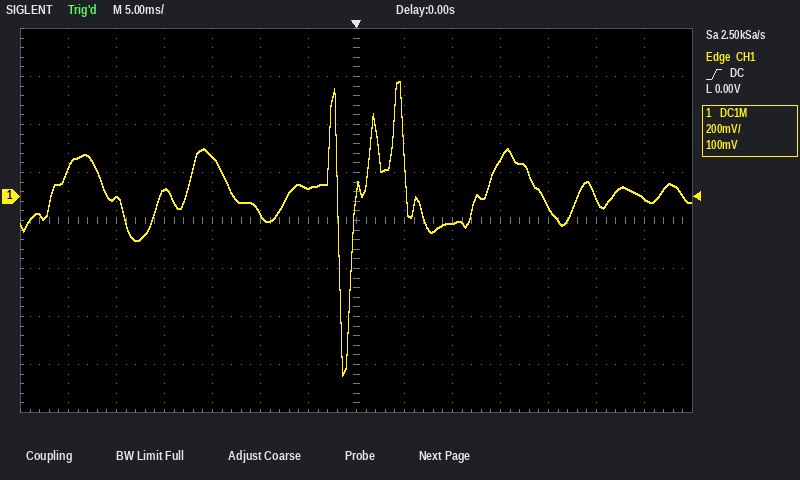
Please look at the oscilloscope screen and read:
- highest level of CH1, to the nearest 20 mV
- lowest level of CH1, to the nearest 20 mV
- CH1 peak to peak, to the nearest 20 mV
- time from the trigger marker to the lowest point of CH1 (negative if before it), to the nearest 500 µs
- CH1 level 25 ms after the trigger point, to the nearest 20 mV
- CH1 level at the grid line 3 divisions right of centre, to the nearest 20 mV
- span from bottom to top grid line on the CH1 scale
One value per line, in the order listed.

480 mV
-740 mV
1.22 V
-1.5 ms
0 mV
160 mV
1.6 V
